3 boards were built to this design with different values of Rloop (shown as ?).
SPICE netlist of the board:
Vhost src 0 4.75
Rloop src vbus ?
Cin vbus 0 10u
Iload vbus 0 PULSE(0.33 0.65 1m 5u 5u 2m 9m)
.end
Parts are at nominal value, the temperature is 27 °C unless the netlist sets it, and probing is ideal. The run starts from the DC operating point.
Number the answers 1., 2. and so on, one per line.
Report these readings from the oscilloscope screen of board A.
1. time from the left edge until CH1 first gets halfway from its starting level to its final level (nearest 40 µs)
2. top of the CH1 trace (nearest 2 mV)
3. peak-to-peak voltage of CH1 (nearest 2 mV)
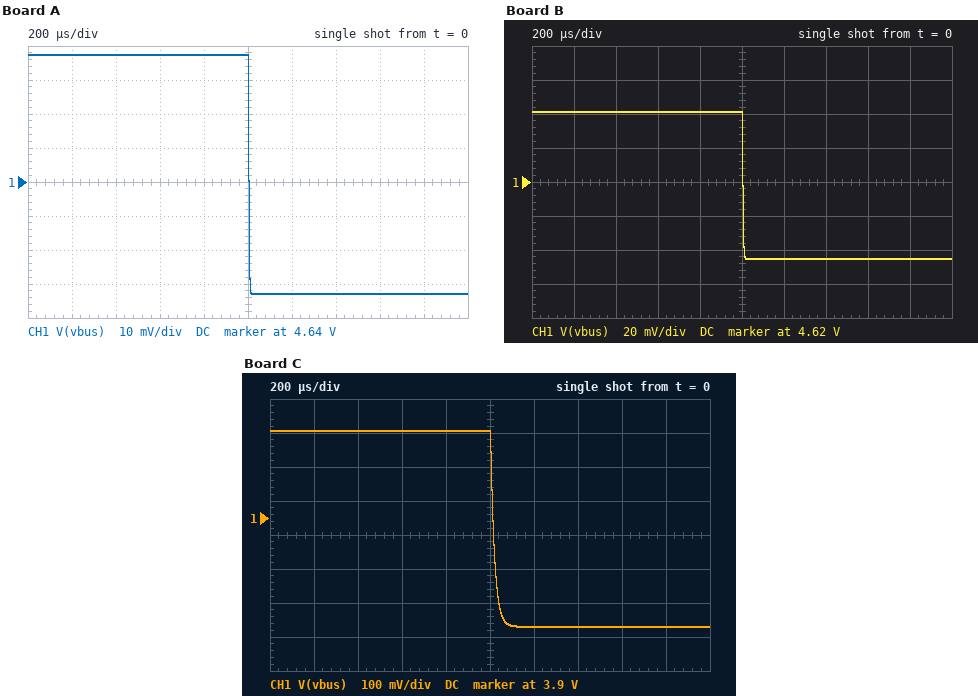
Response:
1. 1.00 ms
2. 4.678 V
3. 70 mV
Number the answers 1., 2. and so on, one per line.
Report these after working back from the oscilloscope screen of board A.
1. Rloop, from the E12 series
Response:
1. 0.22 Ω
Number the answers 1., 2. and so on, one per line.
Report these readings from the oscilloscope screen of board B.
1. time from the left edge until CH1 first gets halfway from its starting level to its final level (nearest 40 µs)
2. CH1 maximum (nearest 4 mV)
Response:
1. 1.00 ms
2. 4.660 V
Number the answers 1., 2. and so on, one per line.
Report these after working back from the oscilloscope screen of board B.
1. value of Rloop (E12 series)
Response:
1. 0.27 Ω
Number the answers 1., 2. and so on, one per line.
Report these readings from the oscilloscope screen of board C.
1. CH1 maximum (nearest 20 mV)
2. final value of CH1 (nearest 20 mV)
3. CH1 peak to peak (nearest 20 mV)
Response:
1. 4.16 V
2. 3.58 V
3. 580 mV
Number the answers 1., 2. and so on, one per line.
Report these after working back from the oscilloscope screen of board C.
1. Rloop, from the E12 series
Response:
1. 1.8 Ω
